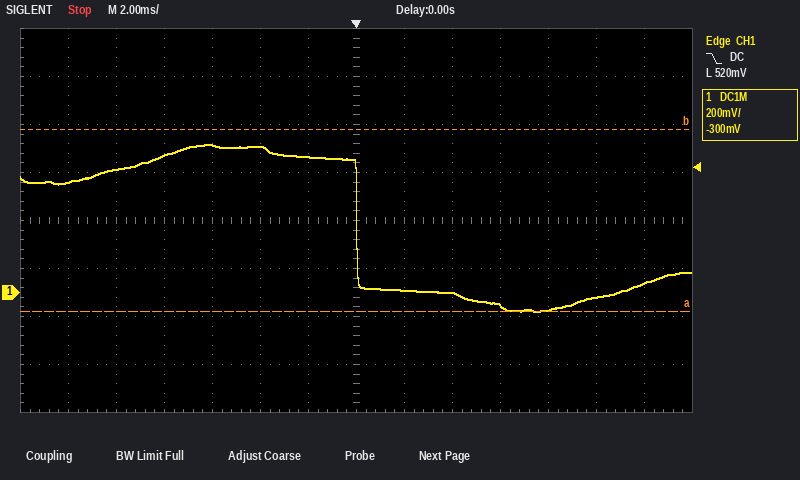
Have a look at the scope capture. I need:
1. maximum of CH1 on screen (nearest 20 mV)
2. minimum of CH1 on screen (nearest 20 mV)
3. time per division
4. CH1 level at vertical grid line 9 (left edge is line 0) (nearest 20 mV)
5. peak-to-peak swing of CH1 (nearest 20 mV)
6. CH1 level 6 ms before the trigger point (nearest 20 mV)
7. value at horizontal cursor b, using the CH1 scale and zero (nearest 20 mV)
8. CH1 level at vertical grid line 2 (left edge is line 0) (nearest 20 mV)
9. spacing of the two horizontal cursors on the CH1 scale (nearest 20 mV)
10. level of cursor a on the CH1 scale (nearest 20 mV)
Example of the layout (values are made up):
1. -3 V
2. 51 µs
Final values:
1. 620 mV
2. -80 mV
3. 2 ms
4. 0 mV
5. 700 mV
6. 620 mV
7. 680 mV
8. 520 mV
9. 760 mV
10. -80 mV
